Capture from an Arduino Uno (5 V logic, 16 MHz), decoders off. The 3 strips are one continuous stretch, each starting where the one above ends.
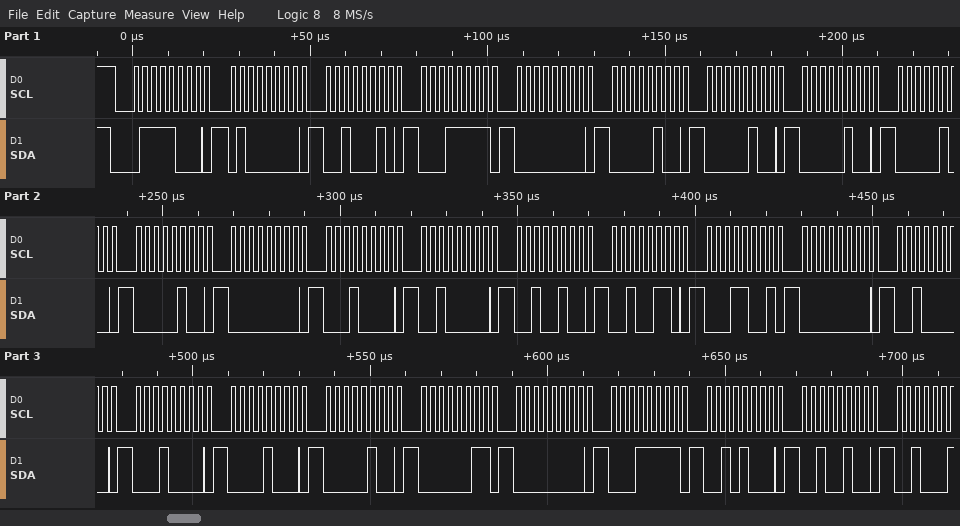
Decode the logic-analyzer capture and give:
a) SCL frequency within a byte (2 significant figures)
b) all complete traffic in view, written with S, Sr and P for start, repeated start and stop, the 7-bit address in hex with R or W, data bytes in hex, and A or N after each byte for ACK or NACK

400 kHz
S 3CW A 40 A 22 A 1F A 00 A 04 A 04 A 04 A 04 A 04 A 00 A 10 A 20 A 24 A 26 A 19 A 00 A 20 A 10 A 08 A 04 A 03 A 00 A 1F A 28 A 24 A
